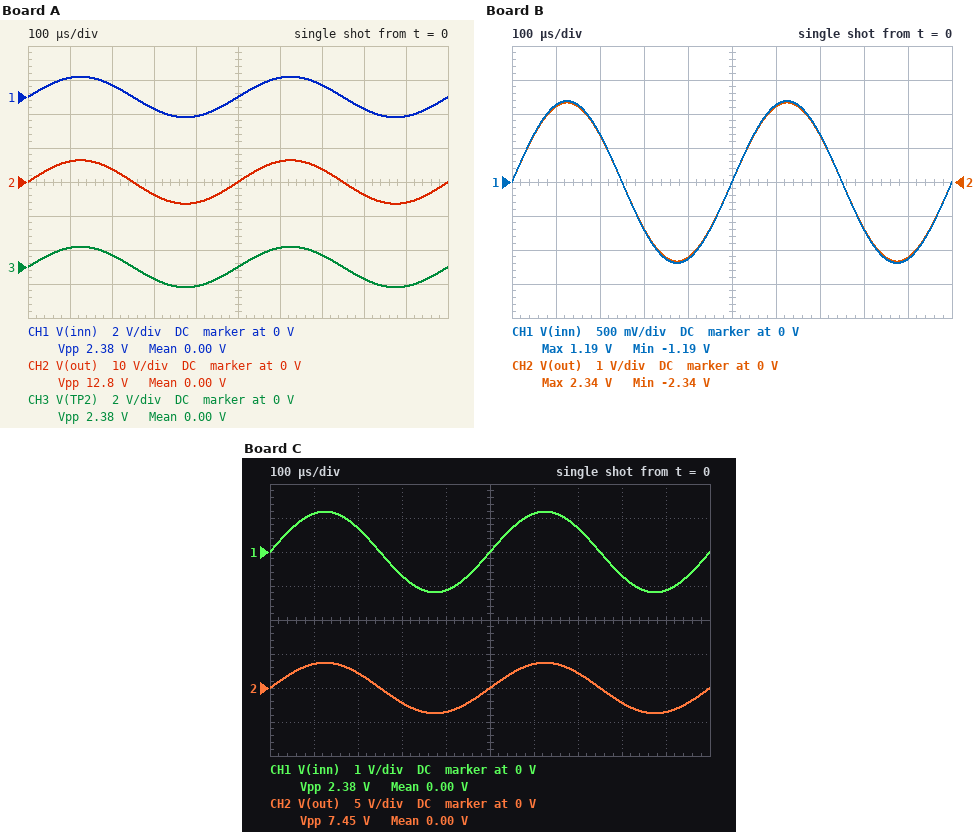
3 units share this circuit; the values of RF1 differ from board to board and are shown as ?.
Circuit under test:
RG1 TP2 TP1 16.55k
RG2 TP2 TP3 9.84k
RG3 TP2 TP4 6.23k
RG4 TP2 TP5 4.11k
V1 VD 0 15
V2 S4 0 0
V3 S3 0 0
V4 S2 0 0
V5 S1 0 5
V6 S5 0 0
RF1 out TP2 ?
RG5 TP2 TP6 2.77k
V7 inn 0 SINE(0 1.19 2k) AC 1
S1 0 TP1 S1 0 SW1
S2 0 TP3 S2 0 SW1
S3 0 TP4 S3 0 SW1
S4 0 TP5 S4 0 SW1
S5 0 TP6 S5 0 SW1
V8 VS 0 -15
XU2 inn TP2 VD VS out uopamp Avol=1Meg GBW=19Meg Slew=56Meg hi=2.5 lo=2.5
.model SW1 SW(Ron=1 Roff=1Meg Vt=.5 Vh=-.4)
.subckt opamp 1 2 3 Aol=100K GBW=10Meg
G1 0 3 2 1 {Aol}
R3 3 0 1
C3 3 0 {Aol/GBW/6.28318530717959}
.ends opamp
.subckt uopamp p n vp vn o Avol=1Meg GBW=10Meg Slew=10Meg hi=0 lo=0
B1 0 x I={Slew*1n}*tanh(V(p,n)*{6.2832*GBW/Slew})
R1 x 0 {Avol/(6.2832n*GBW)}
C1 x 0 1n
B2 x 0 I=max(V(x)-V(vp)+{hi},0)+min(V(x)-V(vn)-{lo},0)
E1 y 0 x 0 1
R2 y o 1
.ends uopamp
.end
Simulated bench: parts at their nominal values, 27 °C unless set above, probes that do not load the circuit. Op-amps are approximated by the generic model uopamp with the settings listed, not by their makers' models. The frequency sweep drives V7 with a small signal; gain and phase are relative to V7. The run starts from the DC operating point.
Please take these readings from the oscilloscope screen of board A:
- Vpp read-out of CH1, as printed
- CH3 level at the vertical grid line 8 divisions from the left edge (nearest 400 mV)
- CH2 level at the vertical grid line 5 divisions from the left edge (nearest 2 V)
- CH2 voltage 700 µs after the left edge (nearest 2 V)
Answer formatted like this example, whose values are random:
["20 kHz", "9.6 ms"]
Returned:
["2.38 V", "-800 mV", "0 V", "4 V"]
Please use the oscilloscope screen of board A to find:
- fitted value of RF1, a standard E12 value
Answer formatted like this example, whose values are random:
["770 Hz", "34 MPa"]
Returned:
["68 kΩ"]
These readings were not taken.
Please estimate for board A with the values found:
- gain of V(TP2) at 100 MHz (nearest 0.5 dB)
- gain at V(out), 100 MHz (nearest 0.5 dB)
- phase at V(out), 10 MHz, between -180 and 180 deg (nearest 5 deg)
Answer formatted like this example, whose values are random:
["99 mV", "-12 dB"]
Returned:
["-17.0 dB", "-14.5 dB", "-35 deg"]
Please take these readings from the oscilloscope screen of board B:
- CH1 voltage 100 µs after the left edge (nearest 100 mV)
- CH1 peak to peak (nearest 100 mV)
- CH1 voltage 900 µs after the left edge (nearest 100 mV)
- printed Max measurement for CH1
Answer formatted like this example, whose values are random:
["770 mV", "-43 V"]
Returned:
["1.1 V", "2.4 V", "-1.1 V", "1.19 V"]
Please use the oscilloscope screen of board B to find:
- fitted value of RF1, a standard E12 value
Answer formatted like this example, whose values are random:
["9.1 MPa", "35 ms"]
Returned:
["15 kΩ"]
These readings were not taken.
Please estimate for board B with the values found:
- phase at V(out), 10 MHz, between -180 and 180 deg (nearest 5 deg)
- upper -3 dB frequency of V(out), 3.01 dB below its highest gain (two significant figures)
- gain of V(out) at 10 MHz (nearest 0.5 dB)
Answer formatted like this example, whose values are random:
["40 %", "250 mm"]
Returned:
["-30 deg", "18 MHz", "-0.5 dB"]
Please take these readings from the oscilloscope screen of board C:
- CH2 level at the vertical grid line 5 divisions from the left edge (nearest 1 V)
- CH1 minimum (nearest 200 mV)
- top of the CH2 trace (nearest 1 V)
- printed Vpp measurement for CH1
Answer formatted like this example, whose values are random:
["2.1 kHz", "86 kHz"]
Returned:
["0 V", "-1.2 V", "4 V", "2.38 V"]
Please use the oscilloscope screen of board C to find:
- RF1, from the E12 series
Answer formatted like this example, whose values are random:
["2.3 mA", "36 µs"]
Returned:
["33 kΩ"]
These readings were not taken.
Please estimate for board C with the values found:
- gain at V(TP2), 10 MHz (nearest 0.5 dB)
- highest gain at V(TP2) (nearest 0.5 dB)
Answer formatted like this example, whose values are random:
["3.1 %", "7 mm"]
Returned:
["-1.5 dB", "0 dB"]
